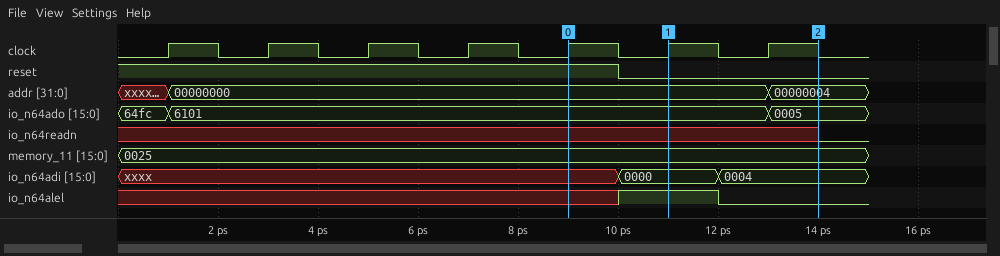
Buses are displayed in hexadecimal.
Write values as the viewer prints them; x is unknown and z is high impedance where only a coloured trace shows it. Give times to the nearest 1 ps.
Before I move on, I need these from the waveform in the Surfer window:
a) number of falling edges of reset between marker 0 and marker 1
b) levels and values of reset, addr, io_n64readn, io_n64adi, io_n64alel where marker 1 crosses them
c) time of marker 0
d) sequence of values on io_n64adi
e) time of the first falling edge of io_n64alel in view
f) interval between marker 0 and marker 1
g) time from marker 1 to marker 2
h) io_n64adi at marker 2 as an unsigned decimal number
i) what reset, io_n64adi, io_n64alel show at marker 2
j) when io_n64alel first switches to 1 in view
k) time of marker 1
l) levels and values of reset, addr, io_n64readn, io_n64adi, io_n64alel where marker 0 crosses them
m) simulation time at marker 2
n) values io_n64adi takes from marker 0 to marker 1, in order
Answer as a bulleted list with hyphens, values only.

- 1
- reset=0, addr=00000000, io_n64readn=x, io_n64adi=0000, io_n64alel=1
- 9 ps
- xxxx, 0000, 0004
- 12 ps
- 2 ps
- 3 ps
- 4
- reset=0, io_n64adi=0004, io_n64alel=0
- 10 ps
- 11 ps
- reset=1, addr=00000000, io_n64readn=x, io_n64adi=xxxx, io_n64alel=x
- 14 ps
- xxxx, 0000
